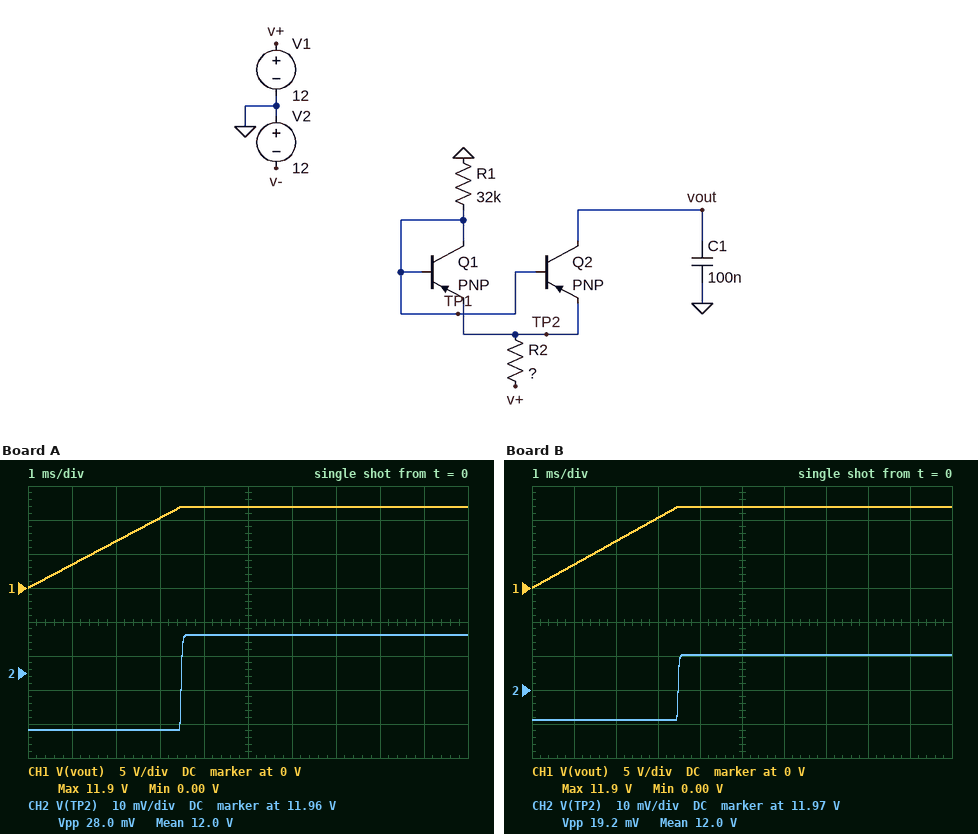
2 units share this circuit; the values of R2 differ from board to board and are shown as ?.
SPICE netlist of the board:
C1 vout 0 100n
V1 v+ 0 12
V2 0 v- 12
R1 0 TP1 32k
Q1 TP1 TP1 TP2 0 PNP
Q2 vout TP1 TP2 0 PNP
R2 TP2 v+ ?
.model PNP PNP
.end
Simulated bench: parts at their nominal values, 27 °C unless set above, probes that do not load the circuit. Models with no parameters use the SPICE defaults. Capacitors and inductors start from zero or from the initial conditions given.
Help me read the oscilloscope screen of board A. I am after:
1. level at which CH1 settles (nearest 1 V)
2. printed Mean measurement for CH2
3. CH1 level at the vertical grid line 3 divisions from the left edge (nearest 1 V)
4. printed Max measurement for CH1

12 V
12.0 V
10 V
11.9 V
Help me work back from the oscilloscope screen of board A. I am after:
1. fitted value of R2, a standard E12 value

82 Ω
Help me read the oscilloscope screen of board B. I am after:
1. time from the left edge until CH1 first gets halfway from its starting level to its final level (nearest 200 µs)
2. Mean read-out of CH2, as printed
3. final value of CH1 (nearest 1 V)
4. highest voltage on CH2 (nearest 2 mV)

1.8 ms
12.0 V
12 V
11.980 V
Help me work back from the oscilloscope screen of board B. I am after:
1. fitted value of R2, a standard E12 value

56 Ω
